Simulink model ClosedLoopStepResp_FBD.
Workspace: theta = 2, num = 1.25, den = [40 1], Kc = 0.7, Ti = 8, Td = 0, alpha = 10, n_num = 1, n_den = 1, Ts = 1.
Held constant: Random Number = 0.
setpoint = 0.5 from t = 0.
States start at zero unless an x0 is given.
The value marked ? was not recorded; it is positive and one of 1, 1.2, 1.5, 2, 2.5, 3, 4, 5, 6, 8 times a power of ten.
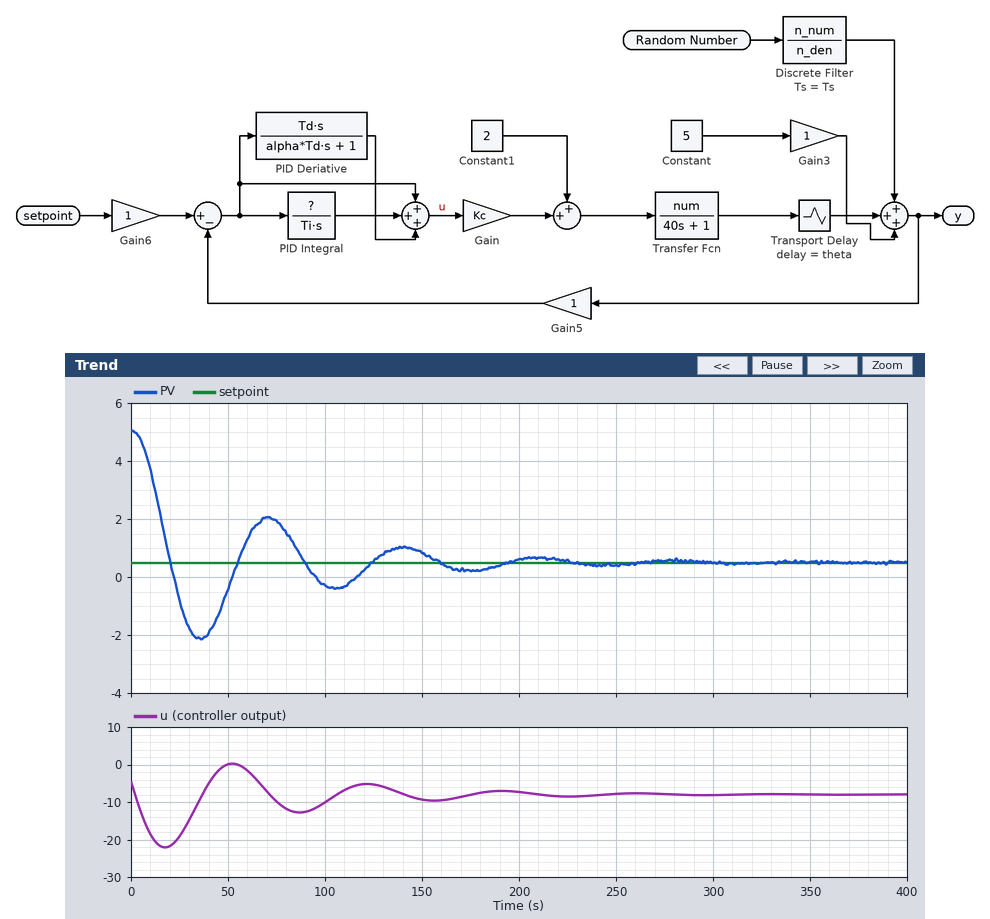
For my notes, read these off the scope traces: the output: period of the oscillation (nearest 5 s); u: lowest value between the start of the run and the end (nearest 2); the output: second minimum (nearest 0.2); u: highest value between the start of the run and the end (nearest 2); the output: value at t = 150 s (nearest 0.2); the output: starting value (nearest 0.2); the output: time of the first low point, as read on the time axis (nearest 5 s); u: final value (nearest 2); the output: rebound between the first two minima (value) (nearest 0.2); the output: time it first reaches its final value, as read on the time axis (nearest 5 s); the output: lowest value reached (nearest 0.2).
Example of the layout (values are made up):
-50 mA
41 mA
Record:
70 s
-22
-0.4
0
0.8
5.0
35 s
-8
2.0
20 s
-2.2
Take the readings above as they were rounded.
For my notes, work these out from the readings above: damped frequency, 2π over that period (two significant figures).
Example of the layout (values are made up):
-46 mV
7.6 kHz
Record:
0.090 rad/s
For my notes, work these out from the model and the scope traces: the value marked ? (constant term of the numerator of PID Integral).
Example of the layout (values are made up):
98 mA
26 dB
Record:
3
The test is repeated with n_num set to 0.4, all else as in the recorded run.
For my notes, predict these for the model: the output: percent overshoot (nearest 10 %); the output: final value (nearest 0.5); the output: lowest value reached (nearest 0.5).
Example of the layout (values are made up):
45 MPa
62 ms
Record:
60 %
0.5
-2.0
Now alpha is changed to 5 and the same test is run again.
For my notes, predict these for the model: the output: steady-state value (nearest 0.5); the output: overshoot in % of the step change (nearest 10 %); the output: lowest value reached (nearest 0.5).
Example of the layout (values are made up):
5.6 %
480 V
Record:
0.5
60 %
-2.0
